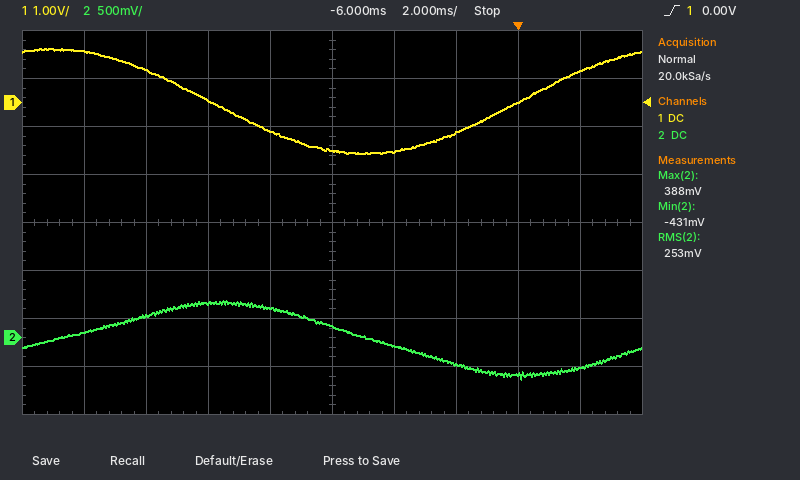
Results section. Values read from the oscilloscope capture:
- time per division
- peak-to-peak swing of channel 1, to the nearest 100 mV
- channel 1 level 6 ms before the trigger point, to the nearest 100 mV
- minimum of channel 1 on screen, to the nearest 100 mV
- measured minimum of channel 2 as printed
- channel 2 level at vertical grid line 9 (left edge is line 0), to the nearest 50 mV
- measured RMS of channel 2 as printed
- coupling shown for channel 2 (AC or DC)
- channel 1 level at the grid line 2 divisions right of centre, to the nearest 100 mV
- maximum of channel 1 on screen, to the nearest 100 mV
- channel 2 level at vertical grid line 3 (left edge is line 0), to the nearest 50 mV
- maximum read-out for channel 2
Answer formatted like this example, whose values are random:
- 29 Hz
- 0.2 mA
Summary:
- 2 ms
- 2.2 V
- -1.0 V
- -1.1 V
- -431 mV
- -300 mV
- 253 mV
- DC
- -600 mV
- 1.1 V
- 350 mV
- 388 mV
